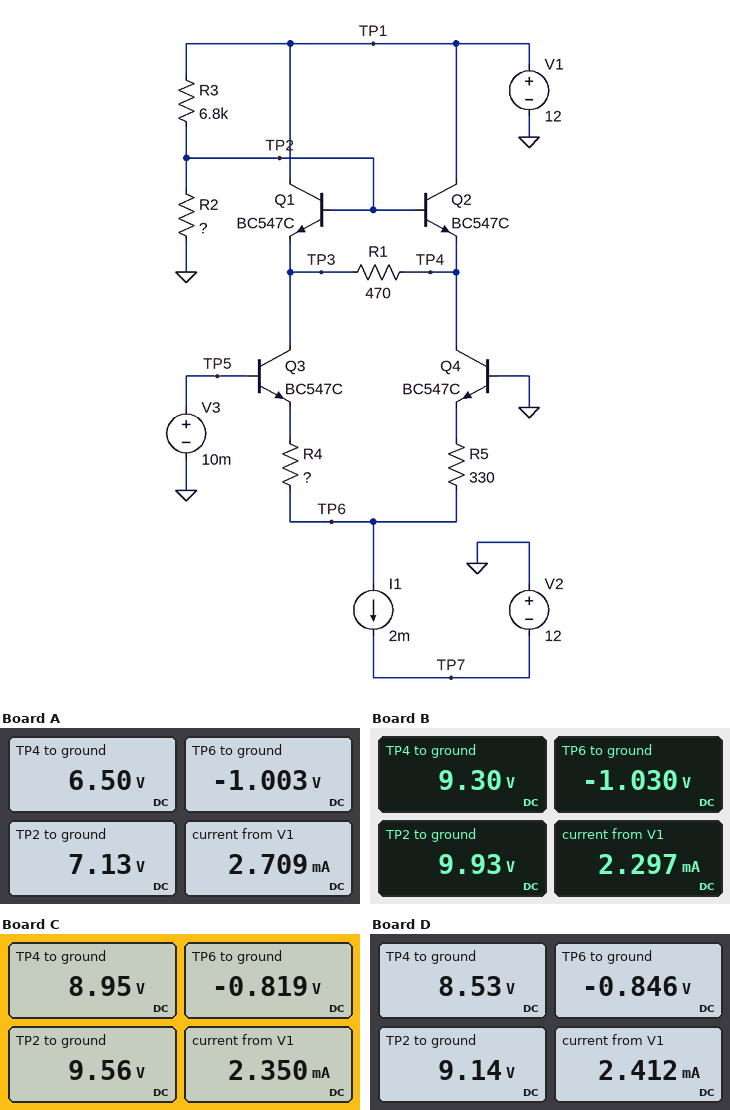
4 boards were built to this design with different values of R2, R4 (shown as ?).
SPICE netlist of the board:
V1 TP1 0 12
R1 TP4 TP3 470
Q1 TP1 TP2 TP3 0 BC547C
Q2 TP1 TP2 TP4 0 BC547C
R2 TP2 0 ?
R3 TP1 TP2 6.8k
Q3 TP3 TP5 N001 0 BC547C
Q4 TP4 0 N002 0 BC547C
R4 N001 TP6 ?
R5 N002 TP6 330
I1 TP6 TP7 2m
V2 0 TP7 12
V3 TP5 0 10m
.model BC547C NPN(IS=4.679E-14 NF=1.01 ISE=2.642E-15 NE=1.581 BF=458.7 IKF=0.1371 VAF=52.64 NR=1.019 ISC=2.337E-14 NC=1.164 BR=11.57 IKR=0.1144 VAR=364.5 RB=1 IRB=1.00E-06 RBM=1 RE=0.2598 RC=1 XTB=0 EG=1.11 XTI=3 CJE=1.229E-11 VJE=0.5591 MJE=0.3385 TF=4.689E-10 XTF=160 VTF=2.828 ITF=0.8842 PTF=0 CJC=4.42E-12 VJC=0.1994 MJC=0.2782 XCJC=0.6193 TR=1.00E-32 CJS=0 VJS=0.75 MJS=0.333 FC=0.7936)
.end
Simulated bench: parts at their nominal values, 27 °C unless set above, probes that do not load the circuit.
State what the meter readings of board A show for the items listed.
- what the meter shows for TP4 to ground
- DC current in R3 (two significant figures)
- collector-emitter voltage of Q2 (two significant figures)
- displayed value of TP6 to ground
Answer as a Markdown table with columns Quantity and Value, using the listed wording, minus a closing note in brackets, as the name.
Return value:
| Quantity | Value |
|---|---|
| what the meter shows for TP4 to ground | 6.50 V |
| DC current in R3 | 720 µA |
| collector-emitter voltage of Q2 | 5.5 V |
| displayed value of TP6 to ground | -1.003 V |
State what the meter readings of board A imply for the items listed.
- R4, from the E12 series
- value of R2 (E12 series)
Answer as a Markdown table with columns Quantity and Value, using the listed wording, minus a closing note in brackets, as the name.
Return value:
| Quantity | Value |
|---|---|
| R4, from the E12 series | 470 Ω |
| value of R2 | 10 kΩ |
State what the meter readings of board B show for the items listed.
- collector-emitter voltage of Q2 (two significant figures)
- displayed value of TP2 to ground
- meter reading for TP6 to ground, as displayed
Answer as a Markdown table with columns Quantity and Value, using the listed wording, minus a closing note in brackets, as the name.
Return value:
| Quantity | Value |
|---|---|
| collector-emitter voltage of Q2 | 2.7 V |
| displayed value of TP2 to ground | 9.93 V |
| meter reading for TP6 to ground, as displayed | -1.030 V |
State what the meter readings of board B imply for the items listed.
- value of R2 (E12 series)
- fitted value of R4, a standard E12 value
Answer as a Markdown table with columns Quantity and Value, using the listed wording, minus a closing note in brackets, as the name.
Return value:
| Quantity | Value |
|---|---|
| value of R2 | 33 kΩ |
| fitted value of R4, a standard E12 value | 560 Ω |
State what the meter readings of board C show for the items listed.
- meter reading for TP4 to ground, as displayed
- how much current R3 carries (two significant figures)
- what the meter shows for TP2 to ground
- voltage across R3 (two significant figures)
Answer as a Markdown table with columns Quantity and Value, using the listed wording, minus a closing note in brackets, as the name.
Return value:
| Quantity | Value |
|---|---|
| meter reading for TP4 to ground, as displayed | 8.95 V |
| how much current R3 carries | 360 µA |
| what the meter shows for TP2 to ground | 9.56 V |
| voltage across R3 | 2.4 V |
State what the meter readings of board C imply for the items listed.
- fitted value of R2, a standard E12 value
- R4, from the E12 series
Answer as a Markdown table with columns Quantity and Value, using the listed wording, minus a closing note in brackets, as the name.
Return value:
| Quantity | Value |
|---|---|
| fitted value of R2, a standard E12 value | 27 kΩ |
| R4, from the E12 series | 150 Ω |
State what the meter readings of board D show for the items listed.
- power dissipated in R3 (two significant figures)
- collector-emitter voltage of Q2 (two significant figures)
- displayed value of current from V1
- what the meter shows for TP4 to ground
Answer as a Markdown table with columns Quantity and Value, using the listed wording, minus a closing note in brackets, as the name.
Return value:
| Quantity | Value |
|---|---|
| power dissipated in R3 | 1.2 mW |
| collector-emitter voltage of Q2 | 3.5 V |
| displayed value of current from V1 | 2.412 mA |
| what the meter shows for TP4 to ground | 8.53 V |
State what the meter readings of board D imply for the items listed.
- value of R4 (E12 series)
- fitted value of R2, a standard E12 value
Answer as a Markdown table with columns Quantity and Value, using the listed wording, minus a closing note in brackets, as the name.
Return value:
| Quantity | Value |
|---|---|
| value of R4 | 180 Ω |
| fitted value of R2, a standard E12 value | 22 kΩ |
